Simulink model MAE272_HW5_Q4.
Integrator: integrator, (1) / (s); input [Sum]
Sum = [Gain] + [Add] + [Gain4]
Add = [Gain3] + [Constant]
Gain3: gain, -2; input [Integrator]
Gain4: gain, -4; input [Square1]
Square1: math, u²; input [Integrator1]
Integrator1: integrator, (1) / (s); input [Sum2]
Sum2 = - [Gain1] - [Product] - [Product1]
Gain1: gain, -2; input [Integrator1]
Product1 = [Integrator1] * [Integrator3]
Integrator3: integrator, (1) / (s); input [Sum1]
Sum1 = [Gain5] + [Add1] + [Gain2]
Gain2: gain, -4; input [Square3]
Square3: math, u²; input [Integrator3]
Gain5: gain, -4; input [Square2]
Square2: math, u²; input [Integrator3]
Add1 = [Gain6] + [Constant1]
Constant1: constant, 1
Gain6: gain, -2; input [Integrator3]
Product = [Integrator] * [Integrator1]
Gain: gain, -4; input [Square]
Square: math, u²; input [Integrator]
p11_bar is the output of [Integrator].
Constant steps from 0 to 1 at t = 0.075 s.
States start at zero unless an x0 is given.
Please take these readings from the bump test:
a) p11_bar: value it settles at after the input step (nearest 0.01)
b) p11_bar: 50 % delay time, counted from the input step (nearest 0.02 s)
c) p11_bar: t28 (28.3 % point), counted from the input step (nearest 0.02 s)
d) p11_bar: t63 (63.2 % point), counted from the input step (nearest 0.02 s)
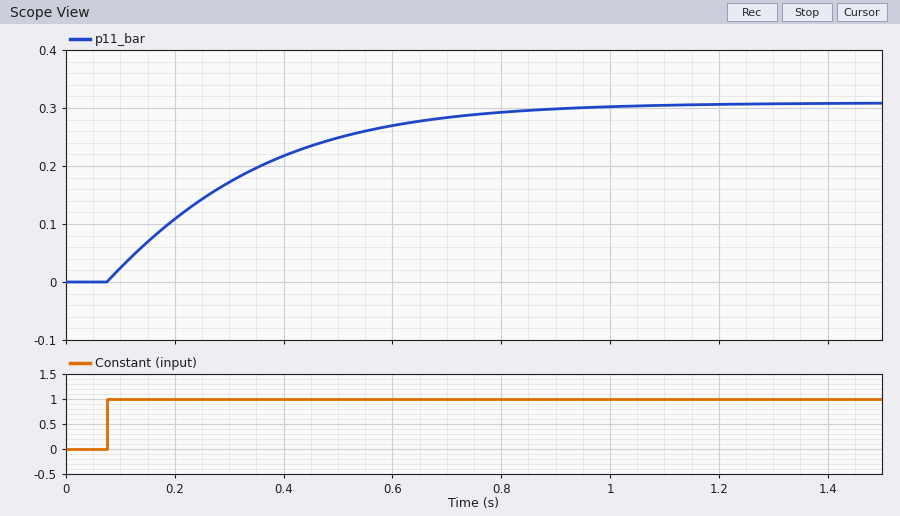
0.31
0.20 s
0.10 s
0.28 s
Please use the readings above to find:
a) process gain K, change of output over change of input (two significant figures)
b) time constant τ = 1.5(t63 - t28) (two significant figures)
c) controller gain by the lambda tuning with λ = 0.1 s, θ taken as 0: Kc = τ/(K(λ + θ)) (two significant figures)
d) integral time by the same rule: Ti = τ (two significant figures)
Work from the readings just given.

0.31
0.27 s
8.7
0.27 s
